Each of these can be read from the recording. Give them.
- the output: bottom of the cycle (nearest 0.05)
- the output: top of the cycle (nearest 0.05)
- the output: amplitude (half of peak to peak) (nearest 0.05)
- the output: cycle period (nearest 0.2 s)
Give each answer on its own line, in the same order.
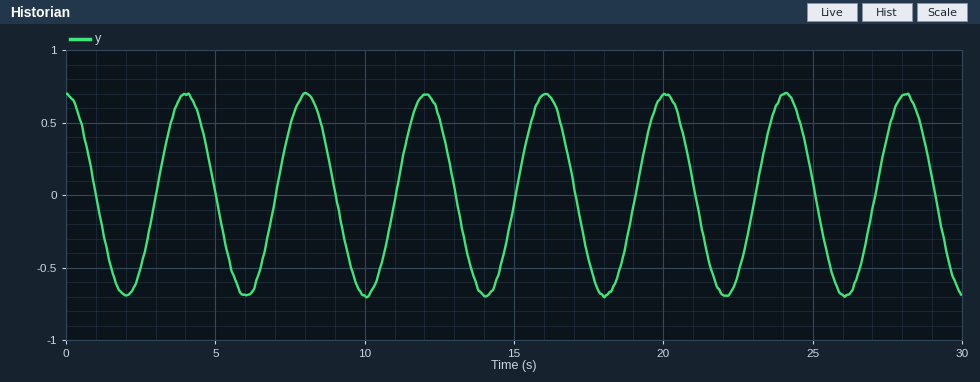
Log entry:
-0.70
0.70
0.70
4.0 s
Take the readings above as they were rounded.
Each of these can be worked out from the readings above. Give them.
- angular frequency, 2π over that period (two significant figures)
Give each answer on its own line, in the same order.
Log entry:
1.6 rad/s
